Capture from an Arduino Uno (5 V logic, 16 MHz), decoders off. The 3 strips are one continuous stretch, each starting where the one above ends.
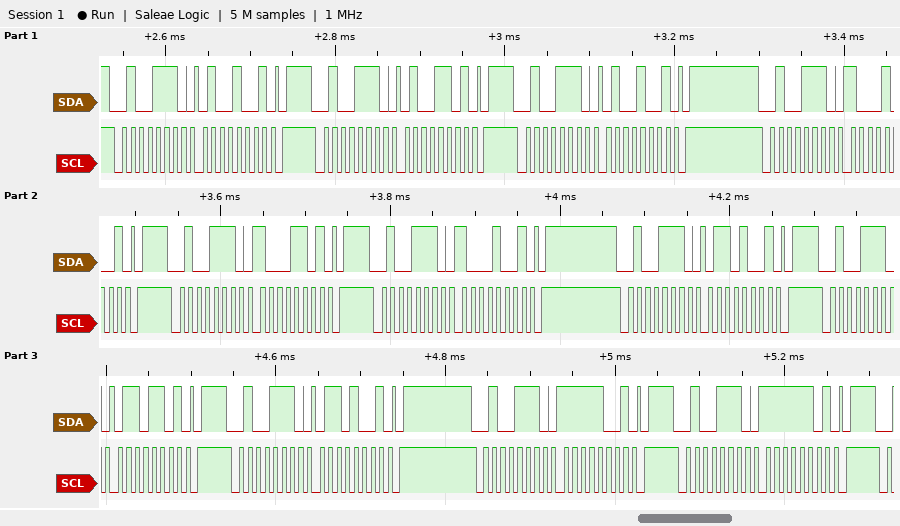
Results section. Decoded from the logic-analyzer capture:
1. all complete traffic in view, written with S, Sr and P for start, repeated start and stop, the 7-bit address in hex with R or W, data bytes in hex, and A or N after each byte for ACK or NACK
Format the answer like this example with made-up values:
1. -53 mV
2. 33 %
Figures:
1. S 27W A 49 A P S 27W A 4D A P S 27W A 49 A P S 27W A 89 A P S 27W A 8D A P S 27W A 89 A P S 27W A 69 A P S 27W A 6D A P S 27W A 69 A P S 27W A F9 A P S 27W A FD A P
